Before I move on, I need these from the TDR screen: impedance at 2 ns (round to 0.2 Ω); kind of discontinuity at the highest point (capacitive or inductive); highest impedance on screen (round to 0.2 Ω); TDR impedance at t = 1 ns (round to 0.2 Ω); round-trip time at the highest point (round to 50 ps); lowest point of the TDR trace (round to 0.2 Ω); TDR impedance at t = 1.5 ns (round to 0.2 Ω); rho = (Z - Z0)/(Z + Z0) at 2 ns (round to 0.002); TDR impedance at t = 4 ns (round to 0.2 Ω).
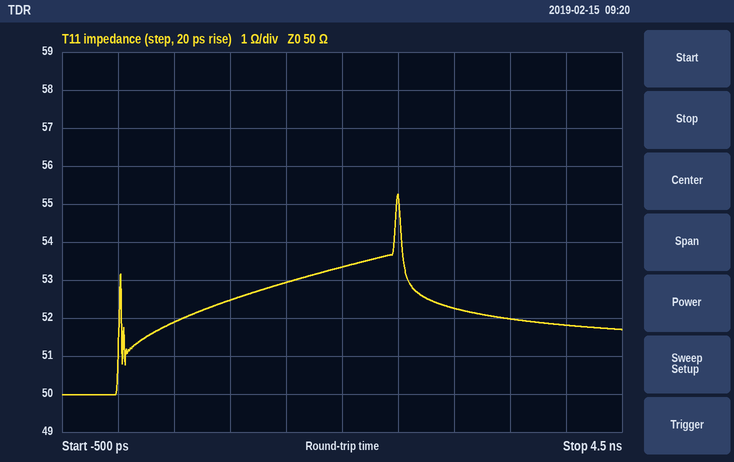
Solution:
53.4 Ω
inductive
55.2 Ω
52.4 Ω
2.50 ns
50.0 Ω
53.0 Ω
+0.032
51.8 Ω
